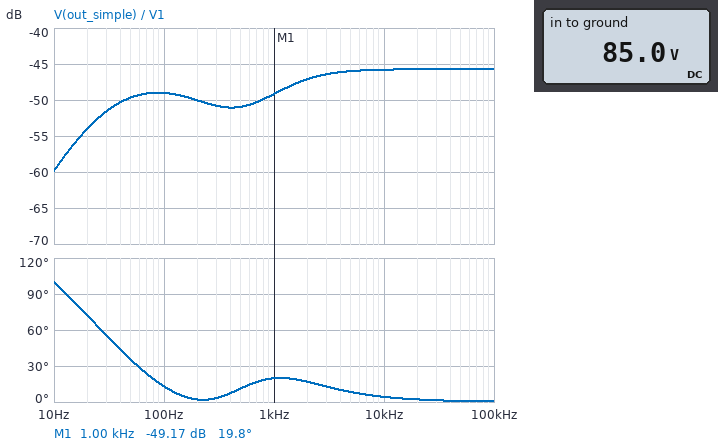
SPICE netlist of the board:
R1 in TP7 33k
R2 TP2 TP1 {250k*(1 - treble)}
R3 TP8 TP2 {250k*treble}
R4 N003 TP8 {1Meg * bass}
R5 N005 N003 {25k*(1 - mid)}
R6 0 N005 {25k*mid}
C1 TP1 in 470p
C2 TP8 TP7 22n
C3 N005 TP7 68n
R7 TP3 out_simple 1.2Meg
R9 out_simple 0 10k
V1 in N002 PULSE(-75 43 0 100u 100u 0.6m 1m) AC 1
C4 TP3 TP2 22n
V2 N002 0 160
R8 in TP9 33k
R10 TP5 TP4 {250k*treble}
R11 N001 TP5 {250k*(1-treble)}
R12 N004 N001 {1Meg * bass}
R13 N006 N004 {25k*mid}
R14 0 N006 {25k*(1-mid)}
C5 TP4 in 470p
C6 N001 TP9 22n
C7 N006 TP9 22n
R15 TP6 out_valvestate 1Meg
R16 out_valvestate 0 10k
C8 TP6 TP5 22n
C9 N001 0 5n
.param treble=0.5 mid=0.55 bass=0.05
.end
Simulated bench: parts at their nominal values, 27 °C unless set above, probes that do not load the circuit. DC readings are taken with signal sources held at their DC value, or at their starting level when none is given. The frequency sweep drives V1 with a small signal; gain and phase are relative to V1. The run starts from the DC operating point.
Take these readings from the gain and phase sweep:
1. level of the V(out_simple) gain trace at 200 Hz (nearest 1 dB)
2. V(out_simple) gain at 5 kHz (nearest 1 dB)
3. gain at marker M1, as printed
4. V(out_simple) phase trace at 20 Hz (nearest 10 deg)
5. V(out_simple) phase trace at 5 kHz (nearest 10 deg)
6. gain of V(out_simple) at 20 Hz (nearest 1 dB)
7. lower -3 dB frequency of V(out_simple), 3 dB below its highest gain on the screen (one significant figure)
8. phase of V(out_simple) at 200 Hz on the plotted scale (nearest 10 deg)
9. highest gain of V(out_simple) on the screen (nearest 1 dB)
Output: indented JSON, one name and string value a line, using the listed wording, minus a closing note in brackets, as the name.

{
  "level of the V(out_simple) gain trace at 200 Hz": "-50 dB",
  "V(out_simple) gain at 5 kHz": "-46 dB",
  "gain at marker M1, as printed": "-49.17 dB",
  "V(out_simple) phase trace at 20 Hz": "70 deg",
  "V(out_simple) phase trace at 5 kHz": "10 deg",
  "gain of V(out_simple) at 20 Hz": "-54 dB",
  "lower -3 dB frequency of V(out_simple), 3 dB below its highest gain on the screen": "1 kHz",
  "phase of V(out_simple) at 200 Hz on the plotted scale": "0 deg",
  "highest gain of V(out_simple) on the screen": "-46 dB"
}
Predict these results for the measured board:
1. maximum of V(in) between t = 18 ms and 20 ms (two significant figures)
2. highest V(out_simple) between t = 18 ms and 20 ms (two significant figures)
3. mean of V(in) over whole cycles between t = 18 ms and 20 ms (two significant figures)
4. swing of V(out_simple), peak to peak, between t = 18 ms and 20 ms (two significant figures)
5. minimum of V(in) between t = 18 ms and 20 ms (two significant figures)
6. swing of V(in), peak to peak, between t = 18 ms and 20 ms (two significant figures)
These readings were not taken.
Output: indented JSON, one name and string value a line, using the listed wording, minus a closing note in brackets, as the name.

{
  "maximum of V(in) between t = 18 ms and 20 ms": "200 V",
  "highest V(out_simple) between t = 18 ms and 20 ms": "250 mV",
  "mean of V(in) over whole cycles between t = 18 ms and 20 ms": "170 V",
  "swing of V(out_simple), peak to peak, between t = 18 ms and 20 ms": "690 mV",
  "minimum of V(in) between t = 18 ms and 20 ms": "85 V",
  "swing of V(in), peak to peak, between t = 18 ms and 20 ms": "120 V"
}
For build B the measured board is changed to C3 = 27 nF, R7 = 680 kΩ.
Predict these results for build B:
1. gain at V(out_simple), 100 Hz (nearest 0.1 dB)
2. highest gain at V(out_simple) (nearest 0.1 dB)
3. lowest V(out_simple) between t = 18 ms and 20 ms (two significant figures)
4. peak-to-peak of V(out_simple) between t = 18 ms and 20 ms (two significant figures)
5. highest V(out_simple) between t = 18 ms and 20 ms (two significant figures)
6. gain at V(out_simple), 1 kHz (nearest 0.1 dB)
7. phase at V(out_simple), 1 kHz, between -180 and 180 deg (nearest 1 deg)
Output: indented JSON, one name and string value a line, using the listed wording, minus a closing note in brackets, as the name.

{
  "gain at V(out_simple), 100 Hz": "-43.5 dB",
  "highest gain at V(out_simple)": "-41.2 dB",
  "lowest V(out_simple) between t = 18 ms and 20 ms": "-710 mV",
  "peak-to-peak of V(out_simple) between t = 18 ms and 20 ms": "1.1 V",
  "highest V(out_simple) between t = 18 ms and 20 ms": "400 mV",
  "gain at V(out_simple), 1 kHz": "-44.8 dB",
  "phase at V(out_simple), 1 kHz, between -180 and 180 deg": "16 deg"
}
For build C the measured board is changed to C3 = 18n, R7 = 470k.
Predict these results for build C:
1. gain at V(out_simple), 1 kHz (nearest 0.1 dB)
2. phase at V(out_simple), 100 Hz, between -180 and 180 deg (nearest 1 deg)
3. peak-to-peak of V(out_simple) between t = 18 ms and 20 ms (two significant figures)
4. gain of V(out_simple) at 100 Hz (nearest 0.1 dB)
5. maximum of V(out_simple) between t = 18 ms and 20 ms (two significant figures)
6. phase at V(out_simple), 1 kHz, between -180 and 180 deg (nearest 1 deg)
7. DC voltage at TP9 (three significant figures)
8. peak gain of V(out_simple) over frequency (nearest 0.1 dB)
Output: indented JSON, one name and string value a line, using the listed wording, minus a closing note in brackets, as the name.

{
  "gain at V(out_simple), 1 kHz": "-42.0 dB",
  "phase at V(out_simple), 100 Hz, between -180 and 180 deg": "32 deg",
  "peak-to-peak of V(out_simple) between t = 18 ms and 20 ms": "1.5 V",
  "gain of V(out_simple) at 100 Hz": "-40.8 dB",
  "maximum of V(out_simple) between t = 18 ms and 20 ms": "530 mV",
  "phase at V(out_simple), 1 kHz, between -180 and 180 deg": "13 deg",
  "DC voltage at TP9": "85.0 V",
  "peak gain of V(out_simple) over frequency": "-38.3 dB"
}
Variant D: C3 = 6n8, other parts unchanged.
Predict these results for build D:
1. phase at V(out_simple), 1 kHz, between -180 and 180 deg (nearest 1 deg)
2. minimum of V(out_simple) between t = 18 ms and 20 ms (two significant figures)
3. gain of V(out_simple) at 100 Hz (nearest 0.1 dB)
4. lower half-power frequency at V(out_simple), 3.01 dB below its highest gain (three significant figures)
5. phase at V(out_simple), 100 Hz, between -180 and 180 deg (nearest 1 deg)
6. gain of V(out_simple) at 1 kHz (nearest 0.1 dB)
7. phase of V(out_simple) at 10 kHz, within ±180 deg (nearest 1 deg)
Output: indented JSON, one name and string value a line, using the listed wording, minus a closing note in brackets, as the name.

{
  "phase at V(out_simple), 1 kHz, between -180 and 180 deg": "1 deg",
  "minimum of V(out_simple) between t = 18 ms and 20 ms": "-410 mV",
  "gain of V(out_simple) at 100 Hz": "-47.1 dB",
  "lower half-power frequency at V(out_simple), 3.01 dB below its highest gain": "62.7 Hz",
  "phase at V(out_simple), 100 Hz, between -180 and 180 deg": "34 deg",
  "gain of V(out_simple) at 1 kHz": "-47.4 dB",
  "phase of V(out_simple) at 10 kHz, within ±180 deg": "3 deg"
}
